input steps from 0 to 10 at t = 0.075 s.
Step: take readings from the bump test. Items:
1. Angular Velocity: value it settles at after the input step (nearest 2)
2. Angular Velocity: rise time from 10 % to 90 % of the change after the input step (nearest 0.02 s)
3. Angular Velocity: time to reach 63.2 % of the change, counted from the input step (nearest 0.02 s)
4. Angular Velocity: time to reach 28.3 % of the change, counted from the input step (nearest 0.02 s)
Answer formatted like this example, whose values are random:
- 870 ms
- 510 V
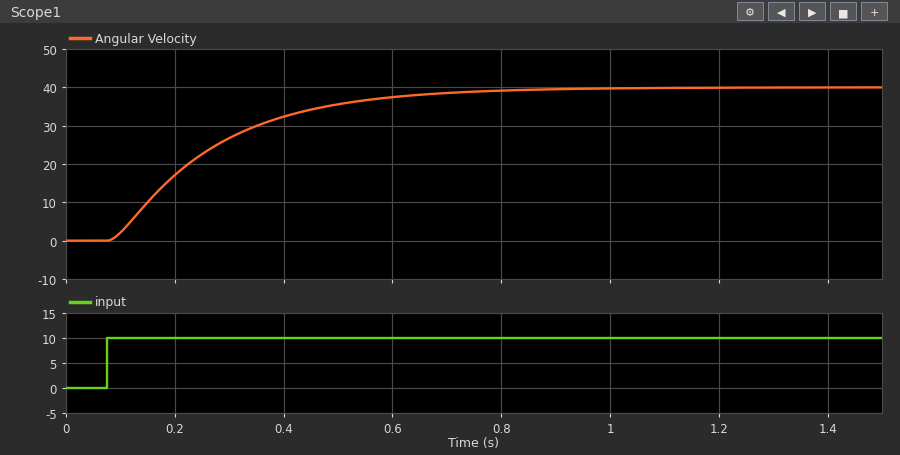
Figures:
- 40
- 0.40 s
- 0.20 s
- 0.08 s
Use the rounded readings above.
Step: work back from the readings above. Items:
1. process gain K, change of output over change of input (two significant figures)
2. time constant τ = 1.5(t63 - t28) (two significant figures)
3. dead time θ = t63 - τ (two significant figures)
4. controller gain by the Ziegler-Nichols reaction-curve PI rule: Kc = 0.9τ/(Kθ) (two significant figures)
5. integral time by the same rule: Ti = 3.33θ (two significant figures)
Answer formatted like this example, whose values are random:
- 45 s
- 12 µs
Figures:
- 4.0
- 0.18 s
- 0.020 s
- 2.0
- 0.067 s
